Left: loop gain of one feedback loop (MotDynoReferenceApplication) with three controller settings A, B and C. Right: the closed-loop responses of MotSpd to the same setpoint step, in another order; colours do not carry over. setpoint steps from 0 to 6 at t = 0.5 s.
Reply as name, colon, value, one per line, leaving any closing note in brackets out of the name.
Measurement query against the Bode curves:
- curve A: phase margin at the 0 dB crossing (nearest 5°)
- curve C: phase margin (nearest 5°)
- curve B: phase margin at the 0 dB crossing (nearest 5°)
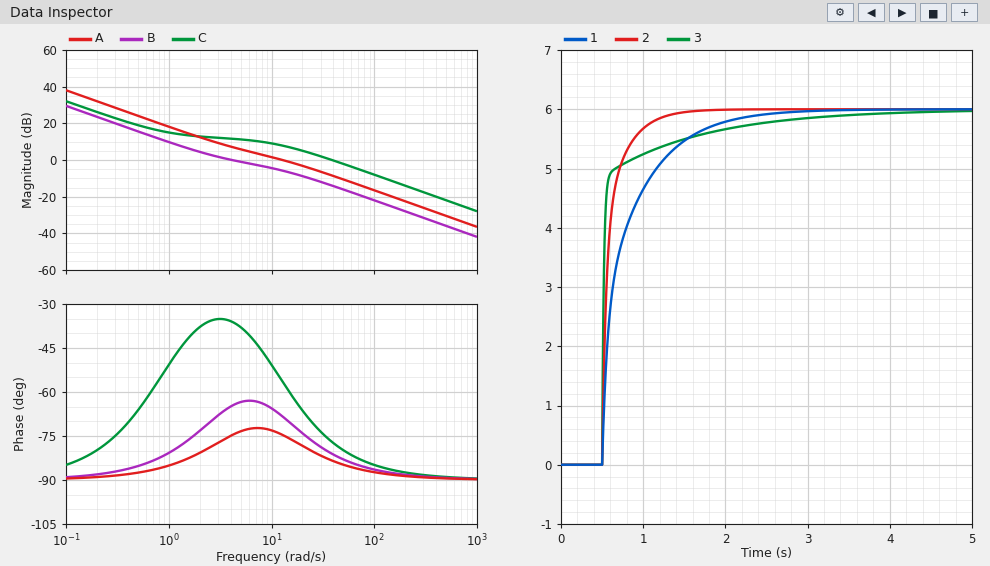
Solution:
curve A: phase margin at the 0 dB crossing: 105°
curve C: phase margin: 105°
curve B: phase margin at the 0 dB crossing: 115°
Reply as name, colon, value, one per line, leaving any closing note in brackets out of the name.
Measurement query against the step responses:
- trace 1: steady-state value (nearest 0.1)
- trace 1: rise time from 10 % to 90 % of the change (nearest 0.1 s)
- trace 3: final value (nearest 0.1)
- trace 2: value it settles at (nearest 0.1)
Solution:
trace 1: steady-state value: 6.0
trace 1: rise time from 10 % to 90 % of the change: 0.9 s
trace 3: final value: 6.0
trace 2: value it settles at: 6.0
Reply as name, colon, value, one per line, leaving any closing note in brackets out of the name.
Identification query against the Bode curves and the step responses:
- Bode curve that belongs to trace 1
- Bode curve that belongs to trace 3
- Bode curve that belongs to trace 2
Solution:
Bode curve that belongs to trace 1: B
Bode curve that belongs to trace 3: C
Bode curve that belongs to trace 2: A
